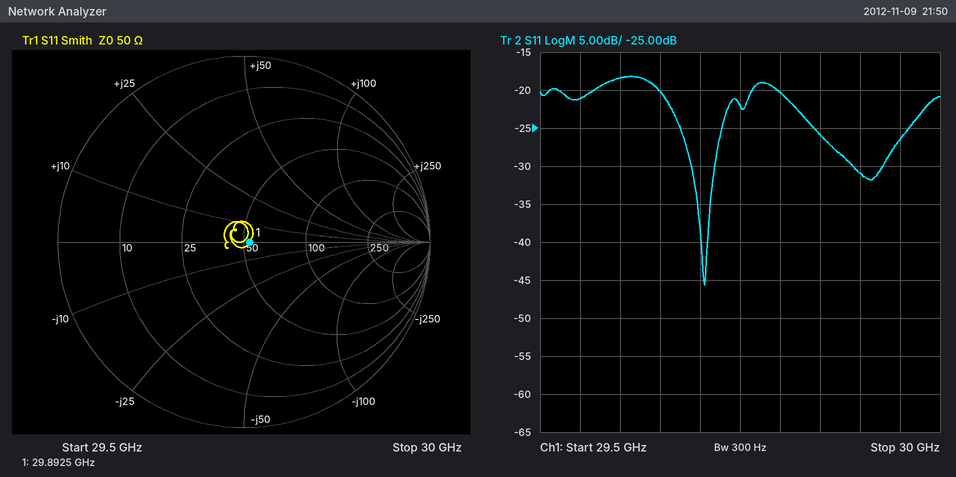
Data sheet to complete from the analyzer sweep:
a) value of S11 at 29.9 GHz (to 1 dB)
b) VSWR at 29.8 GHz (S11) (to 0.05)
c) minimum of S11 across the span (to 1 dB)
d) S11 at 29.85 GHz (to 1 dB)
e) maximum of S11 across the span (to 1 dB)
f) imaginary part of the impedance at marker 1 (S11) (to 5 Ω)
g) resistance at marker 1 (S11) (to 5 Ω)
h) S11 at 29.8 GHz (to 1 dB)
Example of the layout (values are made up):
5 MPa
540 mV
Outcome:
-31 dB
1.20
-46 dB
-26 dB
-18 dB
0 Ω
55 Ω
-20 dB
